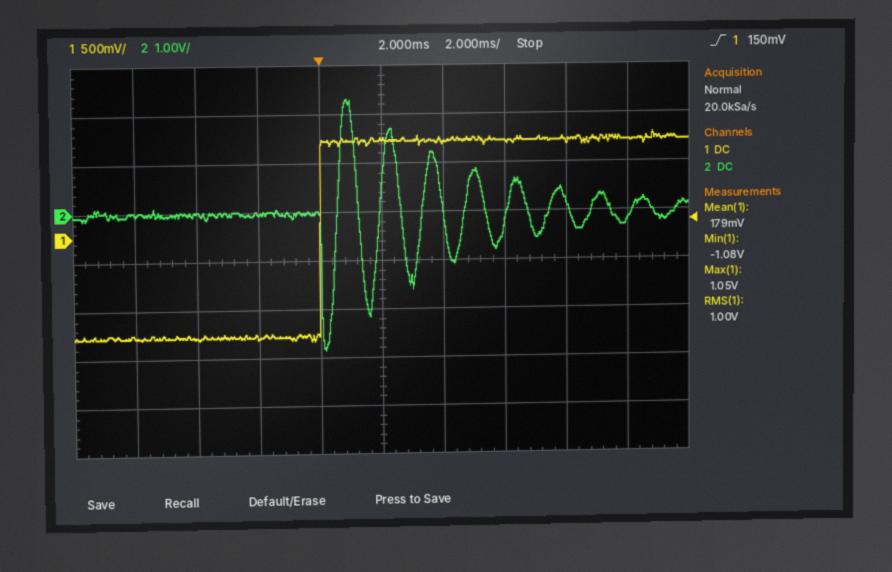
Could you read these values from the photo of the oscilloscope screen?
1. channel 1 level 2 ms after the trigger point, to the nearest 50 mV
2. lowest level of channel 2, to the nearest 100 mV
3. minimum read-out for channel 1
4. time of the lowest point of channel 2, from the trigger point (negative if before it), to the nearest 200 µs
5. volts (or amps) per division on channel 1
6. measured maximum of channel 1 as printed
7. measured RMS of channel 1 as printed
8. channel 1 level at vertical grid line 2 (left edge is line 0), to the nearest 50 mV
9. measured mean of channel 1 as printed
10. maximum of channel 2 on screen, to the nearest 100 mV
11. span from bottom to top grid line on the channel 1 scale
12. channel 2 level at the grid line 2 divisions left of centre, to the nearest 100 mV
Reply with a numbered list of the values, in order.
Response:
1. 1.00 V
2. -2.8 V
3. -1.08 V
4. +200 µs
5. 500 mV
6. 1.05 V
7. 1.00 V
8. -1.05 V
9. 179 mV
10. 2.3 V
11. 4 V
12. 0.0 V
